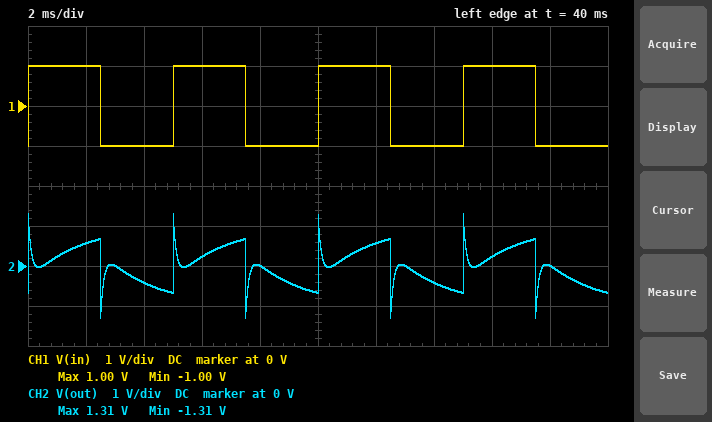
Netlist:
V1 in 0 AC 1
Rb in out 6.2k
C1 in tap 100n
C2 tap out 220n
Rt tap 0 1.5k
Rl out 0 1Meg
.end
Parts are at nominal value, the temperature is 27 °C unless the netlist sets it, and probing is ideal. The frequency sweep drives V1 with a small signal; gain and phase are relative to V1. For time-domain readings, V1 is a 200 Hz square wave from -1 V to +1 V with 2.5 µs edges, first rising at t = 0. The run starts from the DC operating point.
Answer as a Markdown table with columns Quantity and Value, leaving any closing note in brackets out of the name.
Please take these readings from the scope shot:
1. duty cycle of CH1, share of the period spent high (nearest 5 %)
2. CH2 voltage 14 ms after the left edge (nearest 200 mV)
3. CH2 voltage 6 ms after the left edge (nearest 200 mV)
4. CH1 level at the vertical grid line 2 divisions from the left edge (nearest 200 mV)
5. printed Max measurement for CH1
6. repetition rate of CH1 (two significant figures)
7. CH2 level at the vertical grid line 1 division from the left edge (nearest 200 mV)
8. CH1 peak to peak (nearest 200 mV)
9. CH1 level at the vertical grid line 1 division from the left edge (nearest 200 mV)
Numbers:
| Quantity | Value |
|---|---|
| duty cycle of CH1, share of the period spent high | 50 % |
| CH2 voltage 14 ms after the left edge | -400 mV |
| CH2 voltage 6 ms after the left edge | 200 mV |
| CH1 level at the vertical grid line 2 divisions from the left edge | -1.0 V |
| printed Max measurement for CH1 | 1.00 V |
| repetition rate of CH1 | 200 Hz |
| CH2 level at the vertical grid line 1 division from the left edge | 600 mV |
| CH1 peak to peak | 2.0 V |
| CH1 level at the vertical grid line 1 division from the left edge | 1.0 V |
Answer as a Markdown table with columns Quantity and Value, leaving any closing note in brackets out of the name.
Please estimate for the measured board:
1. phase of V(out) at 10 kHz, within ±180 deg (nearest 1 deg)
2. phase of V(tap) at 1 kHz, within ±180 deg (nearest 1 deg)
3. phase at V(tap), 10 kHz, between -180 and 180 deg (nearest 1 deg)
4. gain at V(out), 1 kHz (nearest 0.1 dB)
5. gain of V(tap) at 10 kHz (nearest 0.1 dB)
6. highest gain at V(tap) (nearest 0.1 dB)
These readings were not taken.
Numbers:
| Quantity | Value |
|---|---|
| phase of V(out) at 10 kHz, within ±180 deg | 6 deg |
| phase of V(tap) at 1 kHz, within ±180 deg | 38 deg |
| phase at V(tap), 10 kHz, between -180 and 180 deg | 6 deg |
| gain at V(out), 1 kHz | -4.9 dB |
| gain of V(tap) at 10 kHz | -0.1 dB |
| highest gain at V(tap) | 0 dB |
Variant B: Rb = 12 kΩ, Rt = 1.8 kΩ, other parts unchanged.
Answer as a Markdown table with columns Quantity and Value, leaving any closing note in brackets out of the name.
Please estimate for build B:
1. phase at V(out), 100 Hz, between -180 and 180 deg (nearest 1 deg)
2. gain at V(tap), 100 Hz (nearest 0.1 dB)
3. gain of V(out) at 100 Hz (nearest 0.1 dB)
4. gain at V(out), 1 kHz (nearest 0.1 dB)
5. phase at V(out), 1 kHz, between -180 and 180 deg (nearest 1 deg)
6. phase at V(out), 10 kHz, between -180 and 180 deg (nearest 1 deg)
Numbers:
| Quantity | Value |
|---|---|
| phase at V(out), 100 Hz, between -180 and 180 deg | -44 deg |
| gain at V(tap), 100 Hz | -14.6 dB |
| gain of V(out) at 100 Hz | -7.8 dB |
| gain at V(out), 1 kHz | -3.4 dB |
| phase at V(out), 1 kHz, between -180 and 180 deg | 37 deg |
| phase at V(out), 10 kHz, between -180 and 180 deg | 5 deg |
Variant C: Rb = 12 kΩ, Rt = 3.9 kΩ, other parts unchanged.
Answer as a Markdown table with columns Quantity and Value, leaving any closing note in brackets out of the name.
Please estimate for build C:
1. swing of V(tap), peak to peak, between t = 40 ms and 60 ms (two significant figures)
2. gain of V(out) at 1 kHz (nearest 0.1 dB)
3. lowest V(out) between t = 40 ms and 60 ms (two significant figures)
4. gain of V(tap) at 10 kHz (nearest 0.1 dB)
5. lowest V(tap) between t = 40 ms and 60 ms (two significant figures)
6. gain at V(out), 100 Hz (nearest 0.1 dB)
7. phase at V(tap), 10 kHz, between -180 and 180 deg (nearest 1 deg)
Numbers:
| Quantity | Value |
|---|---|
| swing of V(tap), peak to peak, between t = 40 ms and 60 ms | 3.6 V |
| gain of V(out) at 1 kHz | -1.2 dB |
| lowest V(out) between t = 40 ms and 60 ms | -1.5 V |
| gain of V(tap) at 10 kHz | 0 dB |
| lowest V(tap) between t = 40 ms and 60 ms | -1.8 V |
| gain at V(out), 100 Hz | -8.2 dB |
| phase at V(tap), 10 kHz, between -180 and 180 deg | 2 deg |
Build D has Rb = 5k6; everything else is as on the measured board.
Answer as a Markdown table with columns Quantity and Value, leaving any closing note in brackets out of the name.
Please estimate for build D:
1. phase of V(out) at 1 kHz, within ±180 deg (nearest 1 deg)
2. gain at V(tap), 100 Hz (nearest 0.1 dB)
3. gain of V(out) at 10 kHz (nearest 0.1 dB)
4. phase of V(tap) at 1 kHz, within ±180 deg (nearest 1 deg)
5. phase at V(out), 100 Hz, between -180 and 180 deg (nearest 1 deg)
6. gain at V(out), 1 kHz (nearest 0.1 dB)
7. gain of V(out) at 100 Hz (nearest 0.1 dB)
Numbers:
| Quantity | Value |
|---|---|
| phase of V(out) at 1 kHz, within ±180 deg | 34 deg |
| gain at V(tap), 100 Hz | -13.2 dB |
| gain of V(out) at 10 kHz | -0.1 dB |
| phase of V(tap) at 1 kHz, within ±180 deg | 37 deg |
| phase at V(out), 100 Hz, between -180 and 180 deg | -31 deg |
| gain at V(out), 1 kHz | -5.0 dB |
| gain of V(out) at 100 Hz | -3.3 dB |
